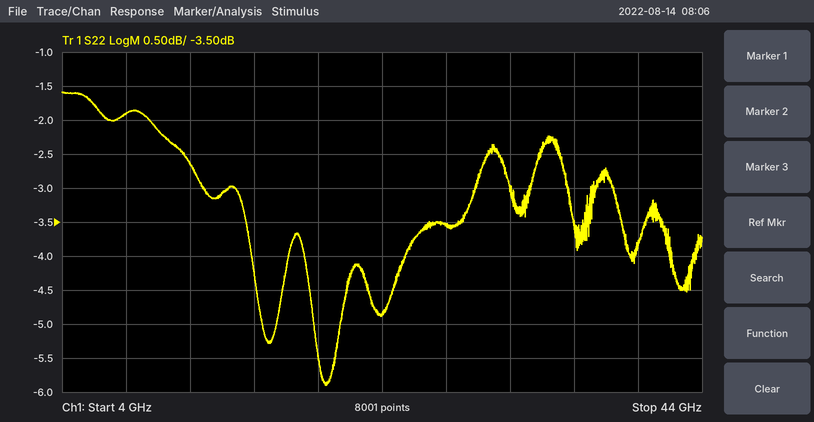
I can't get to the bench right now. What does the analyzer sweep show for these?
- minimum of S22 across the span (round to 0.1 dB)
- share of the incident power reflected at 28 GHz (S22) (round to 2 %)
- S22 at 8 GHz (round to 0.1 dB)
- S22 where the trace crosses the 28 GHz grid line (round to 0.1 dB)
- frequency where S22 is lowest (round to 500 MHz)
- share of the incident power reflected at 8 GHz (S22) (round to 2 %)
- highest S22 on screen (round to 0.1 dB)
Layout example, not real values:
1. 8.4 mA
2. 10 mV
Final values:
1. -5.9 dB
2. 44 %
3. -1.9 dB
4. -3.5 dB
5. 20.5 GHz
6. 64 %
7. -1.6 dB
